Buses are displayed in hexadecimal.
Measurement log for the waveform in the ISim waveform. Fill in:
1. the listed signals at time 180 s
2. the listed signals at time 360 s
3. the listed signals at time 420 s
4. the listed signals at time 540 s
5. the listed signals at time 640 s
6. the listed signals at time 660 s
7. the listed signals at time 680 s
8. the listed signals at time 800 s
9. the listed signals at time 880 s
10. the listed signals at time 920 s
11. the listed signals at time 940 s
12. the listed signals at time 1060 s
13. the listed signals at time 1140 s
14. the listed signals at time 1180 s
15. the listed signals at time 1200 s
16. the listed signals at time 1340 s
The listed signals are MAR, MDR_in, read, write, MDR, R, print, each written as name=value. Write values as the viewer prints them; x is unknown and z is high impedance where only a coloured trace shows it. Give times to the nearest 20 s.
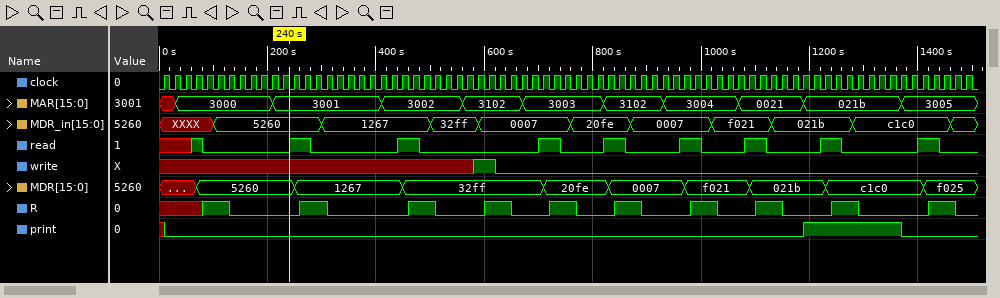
MAR=3000, MDR_in=5260, read=0, write=x, MDR=5260, R=0, print=0
MAR=3001, MDR_in=1267, read=0, write=x, MDR=1267, R=0, print=0
MAR=3002, MDR_in=1267, read=0, write=x, MDR=1267, R=0, print=0
MAR=3002, MDR_in=32ff, read=0, write=x, MDR=32ff, R=0, print=0
MAR=3102, MDR_in=0007, read=0, write=0, MDR=32ff, R=1, print=0
MAR=3102, MDR_in=0007, read=0, write=0, MDR=32ff, R=0, print=0
MAR=3003, MDR_in=0007, read=0, write=0, MDR=32ff, R=0, print=0
MAR=3003, MDR_in=20fe, read=0, write=0, MDR=20fe, R=0, print=0
MAR=3102, MDR_in=0007, read=0, write=0, MDR=0007, R=1, print=0
MAR=3102, MDR_in=0007, read=0, write=0, MDR=0007, R=0, print=0
MAR=3004, MDR_in=0007, read=0, write=0, MDR=0007, R=0, print=0
MAR=3004, MDR_in=f021, read=0, write=0, MDR=f021, R=0, print=0
MAR=0021, MDR_in=021b, read=0, write=0, MDR=021b, R=1, print=0
MAR=0021, MDR_in=021b, read=0, write=0, MDR=021b, R=0, print=0
MAR=021b, MDR_in=021b, read=0, write=0, MDR=021b, R=0, print=1
MAR=021b, MDR_in=c1c0, read=0, write=0, MDR=c1c0, R=0, print=1
